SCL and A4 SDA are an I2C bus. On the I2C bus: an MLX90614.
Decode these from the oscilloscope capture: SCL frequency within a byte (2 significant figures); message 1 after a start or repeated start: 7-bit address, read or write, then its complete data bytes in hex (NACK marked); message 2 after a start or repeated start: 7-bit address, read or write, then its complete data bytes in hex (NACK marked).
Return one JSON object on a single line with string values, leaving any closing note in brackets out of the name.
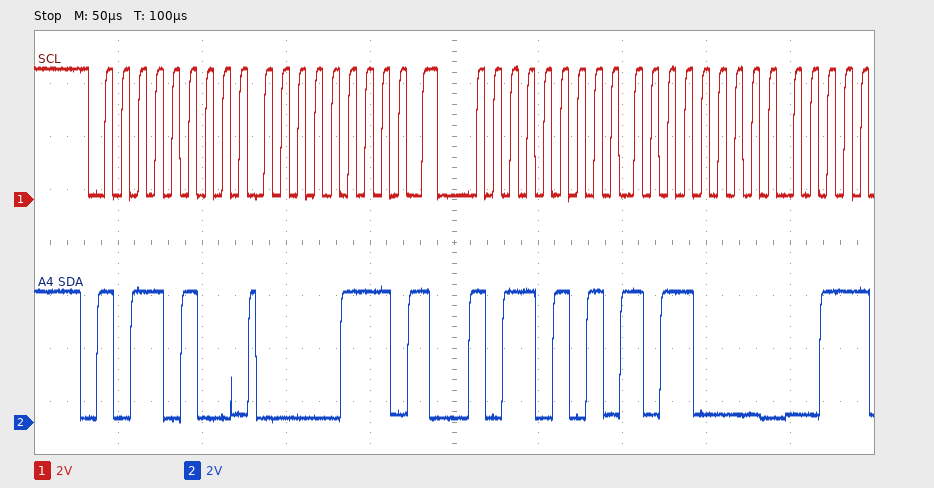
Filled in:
{"SCL frequency within a byte": "100 kHz", "message 1 after a start or repeated start: 7-bit address, read or write, then its complete data bytes in hex": "0x5A write: 07", "message 2 after a start or repeated start: 7-bit address, read or write, then its complete data bytes in hex": "0x5A read: B0"}
